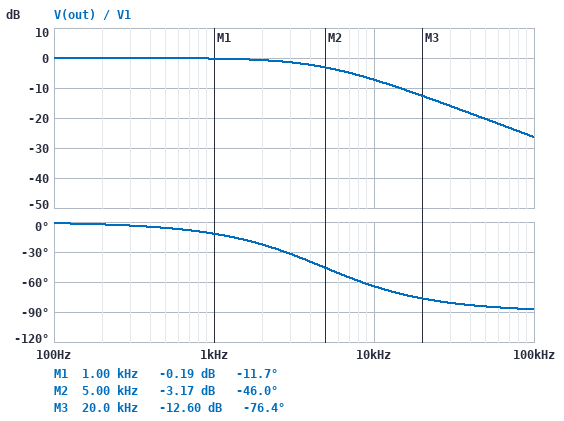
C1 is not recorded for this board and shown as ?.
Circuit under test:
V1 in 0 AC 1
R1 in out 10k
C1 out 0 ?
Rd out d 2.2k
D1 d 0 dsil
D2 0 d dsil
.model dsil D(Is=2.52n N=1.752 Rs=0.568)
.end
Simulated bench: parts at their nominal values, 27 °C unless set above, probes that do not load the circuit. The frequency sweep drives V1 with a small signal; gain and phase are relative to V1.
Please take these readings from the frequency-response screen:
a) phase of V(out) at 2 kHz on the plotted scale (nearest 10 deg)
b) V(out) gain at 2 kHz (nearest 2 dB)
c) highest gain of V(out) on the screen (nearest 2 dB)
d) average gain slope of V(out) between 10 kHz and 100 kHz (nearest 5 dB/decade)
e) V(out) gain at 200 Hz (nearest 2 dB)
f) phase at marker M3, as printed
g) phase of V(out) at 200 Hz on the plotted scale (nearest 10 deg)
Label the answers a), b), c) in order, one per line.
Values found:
a) -20 deg
b) 0 dB
c) 0 dB
d) -20 dB/decade
e) 0 dB
f) -76.4 deg
g) 0 deg
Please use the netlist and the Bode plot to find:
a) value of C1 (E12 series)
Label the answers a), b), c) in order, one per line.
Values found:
a) 3.3 nF
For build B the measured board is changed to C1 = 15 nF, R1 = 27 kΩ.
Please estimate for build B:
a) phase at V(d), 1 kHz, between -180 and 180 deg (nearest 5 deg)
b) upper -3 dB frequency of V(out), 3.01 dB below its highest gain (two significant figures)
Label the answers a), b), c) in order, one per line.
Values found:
a) -70 deg
b) 390 Hz
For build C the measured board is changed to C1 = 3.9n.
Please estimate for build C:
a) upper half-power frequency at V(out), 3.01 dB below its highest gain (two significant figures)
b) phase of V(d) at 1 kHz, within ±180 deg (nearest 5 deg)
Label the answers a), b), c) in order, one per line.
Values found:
a) 4.1 kHz
b) -15 deg
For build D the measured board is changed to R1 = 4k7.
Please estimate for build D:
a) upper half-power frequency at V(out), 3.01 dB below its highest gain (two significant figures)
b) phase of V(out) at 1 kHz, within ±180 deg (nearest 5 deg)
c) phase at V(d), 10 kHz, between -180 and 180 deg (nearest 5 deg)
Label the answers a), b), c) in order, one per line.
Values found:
a) 10 kHz
b) -5 deg
c) -45 deg
